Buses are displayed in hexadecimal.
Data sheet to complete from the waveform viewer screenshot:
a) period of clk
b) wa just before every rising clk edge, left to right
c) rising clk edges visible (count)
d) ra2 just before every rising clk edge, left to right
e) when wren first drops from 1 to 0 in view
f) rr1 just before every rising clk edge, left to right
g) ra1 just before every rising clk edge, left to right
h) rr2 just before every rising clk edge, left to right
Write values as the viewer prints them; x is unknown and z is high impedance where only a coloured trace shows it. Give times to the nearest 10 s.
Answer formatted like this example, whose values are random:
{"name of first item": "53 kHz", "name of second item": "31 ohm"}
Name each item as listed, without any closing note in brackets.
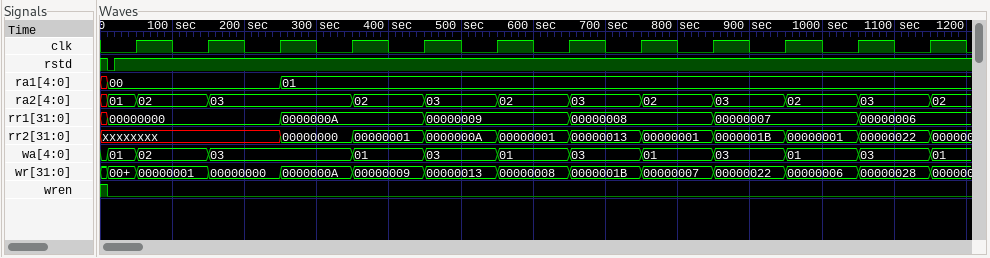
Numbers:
{"period of clk": "100 s", "wa just before every rising clk edge, left to right": "01, 02, 03, 03, 01, 03, 01, 03, 01, 03, 01, 03", "rising clk edges visible": "12", "ra2 just before every rising clk edge, left to right": "01, 02, 03, 03, 02, 03, 02, 03, 02, 03, 02, 03", "when wren first drops from 1 to 0 in view": "10 s", "rr1 just before every rising clk edge, left to right": "00000000, 00000000, 00000000, 0000000A, 0000000A, 00000009, 00000009, 00000008, 00000008, 00000007, 00000007, 00000006", "ra1 just before every rising clk edge, left to right": "00, 00, 00, 01, 01, 01, 01, 01, 01, 01, 01, 01", "rr2 just before every rising clk edge, left to right": "xxxxxxxx, xxxxxxxx, xxxxxxxx, 00000000, 00000001, 0000000A, 00000001, 00000013, 00000001, 0000001B, 00000001, 00000022"}
